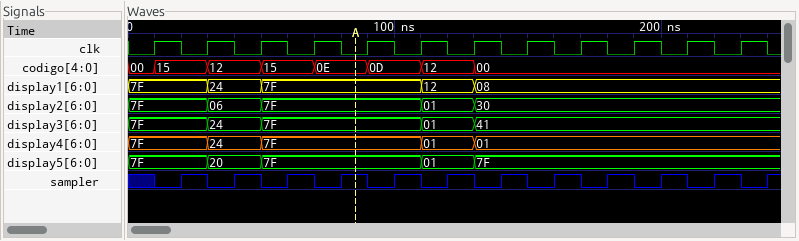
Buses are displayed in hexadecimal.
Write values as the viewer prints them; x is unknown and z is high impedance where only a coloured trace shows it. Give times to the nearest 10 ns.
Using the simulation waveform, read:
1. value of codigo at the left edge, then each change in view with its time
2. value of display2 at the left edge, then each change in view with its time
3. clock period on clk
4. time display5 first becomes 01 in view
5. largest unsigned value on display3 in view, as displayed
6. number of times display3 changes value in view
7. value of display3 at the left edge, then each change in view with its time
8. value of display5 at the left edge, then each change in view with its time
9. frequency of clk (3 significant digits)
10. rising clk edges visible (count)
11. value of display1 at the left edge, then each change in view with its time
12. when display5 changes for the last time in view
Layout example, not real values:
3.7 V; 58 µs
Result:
00, 15 at 10 ns, 12 at 30 ns, 15 at 50 ns, 0E at 70 ns, 0D at 90 ns, 12 at 110 ns, 00 at 130 ns; 7F, 06 at 30 ns, 7F at 50 ns, 01 at 110 ns, 30 at 130 ns; 20 ns; 110 ns; 7F; 4; 7F, 24 at 30 ns, 7F at 50 ns, 01 at 110 ns, 41 at 130 ns; 7F, 20 at 30 ns, 7F at 50 ns, 01 at 110 ns, 7F at 130 ns; 50.0 MHz; 12; 7F, 24 at 30 ns, 7F at 50 ns, 12 at 110 ns, 08 at 130 ns; 130 ns
